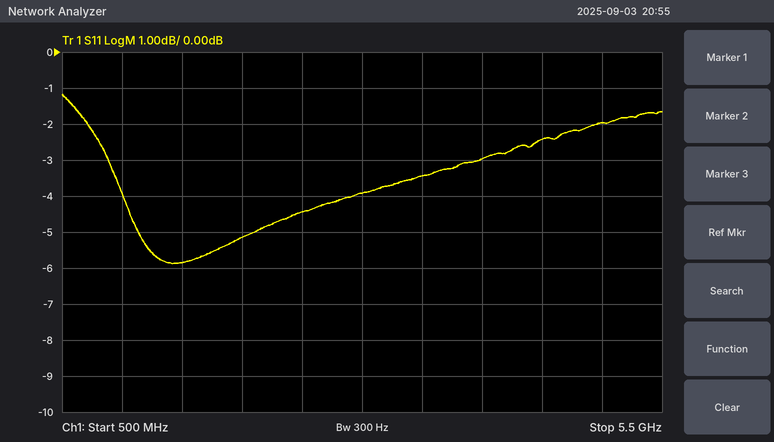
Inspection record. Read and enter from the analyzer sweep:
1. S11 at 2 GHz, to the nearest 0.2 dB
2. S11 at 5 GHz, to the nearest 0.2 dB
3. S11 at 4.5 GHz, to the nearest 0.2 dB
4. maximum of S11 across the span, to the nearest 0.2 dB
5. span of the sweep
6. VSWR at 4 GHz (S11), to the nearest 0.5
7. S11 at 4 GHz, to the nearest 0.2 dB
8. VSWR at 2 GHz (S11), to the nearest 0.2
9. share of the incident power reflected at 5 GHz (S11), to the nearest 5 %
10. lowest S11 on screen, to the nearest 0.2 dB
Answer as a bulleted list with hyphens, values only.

- -5.2 dB
- -2.0 dB
- -2.4 dB
- -1.2 dB
- 5 GHz
- 6.0
- -3.0 dB
- 3.4
- 65 %
- -5.8 dB
